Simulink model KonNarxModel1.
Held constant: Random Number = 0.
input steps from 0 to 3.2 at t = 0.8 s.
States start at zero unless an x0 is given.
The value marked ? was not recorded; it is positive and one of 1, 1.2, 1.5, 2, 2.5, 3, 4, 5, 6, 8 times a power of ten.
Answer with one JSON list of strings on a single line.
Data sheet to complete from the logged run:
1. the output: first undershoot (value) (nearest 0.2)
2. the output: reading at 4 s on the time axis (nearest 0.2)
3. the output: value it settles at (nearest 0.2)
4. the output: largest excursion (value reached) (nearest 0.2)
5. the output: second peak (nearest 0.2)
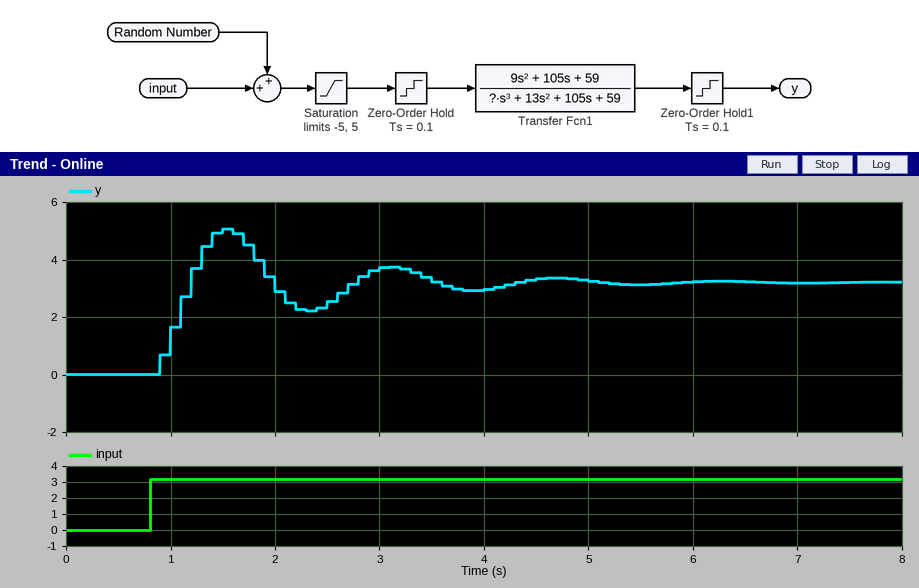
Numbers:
["2.2", "3.0", "3.2", "5.0", "3.8"]
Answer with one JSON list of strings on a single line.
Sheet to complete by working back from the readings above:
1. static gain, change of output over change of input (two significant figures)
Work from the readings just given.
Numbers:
["1.0"]
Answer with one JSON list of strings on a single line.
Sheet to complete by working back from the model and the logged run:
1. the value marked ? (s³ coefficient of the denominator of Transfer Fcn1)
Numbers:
["6"]
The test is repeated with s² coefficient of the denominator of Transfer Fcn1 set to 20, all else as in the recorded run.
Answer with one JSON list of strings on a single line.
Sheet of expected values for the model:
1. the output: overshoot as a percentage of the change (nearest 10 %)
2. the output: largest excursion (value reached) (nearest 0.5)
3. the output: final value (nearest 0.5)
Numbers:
["40 %", "4.5", "3.0"]
